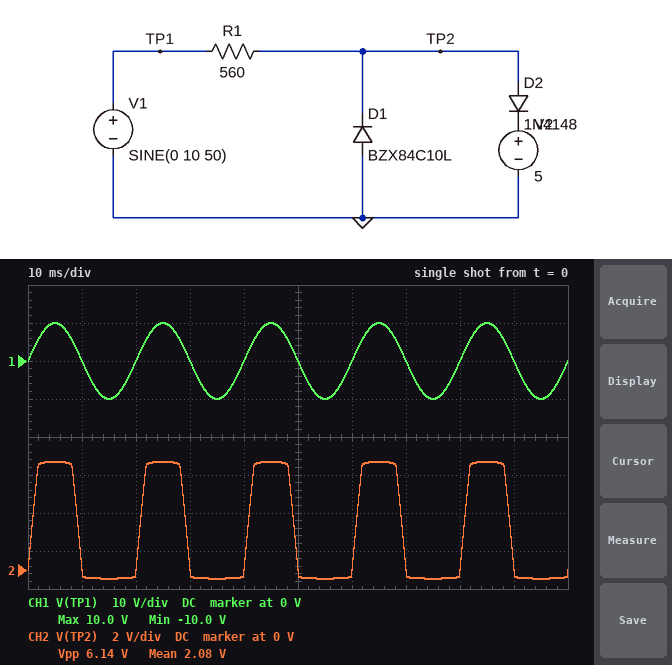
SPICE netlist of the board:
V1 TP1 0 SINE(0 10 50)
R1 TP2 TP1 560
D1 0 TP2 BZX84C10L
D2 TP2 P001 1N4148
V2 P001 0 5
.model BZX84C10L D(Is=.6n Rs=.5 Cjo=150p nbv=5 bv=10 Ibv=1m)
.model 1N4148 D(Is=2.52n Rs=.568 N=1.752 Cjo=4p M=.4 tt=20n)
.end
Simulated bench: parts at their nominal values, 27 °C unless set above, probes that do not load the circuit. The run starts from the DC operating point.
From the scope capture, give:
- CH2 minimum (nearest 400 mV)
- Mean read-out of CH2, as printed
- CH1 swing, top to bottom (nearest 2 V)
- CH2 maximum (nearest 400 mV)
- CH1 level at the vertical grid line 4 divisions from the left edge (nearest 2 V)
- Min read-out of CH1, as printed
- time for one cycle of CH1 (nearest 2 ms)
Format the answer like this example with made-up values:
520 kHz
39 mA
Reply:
-400 mV
2.08 V
20 V
5.6 V
0 V
-10.0 V
20 ms
